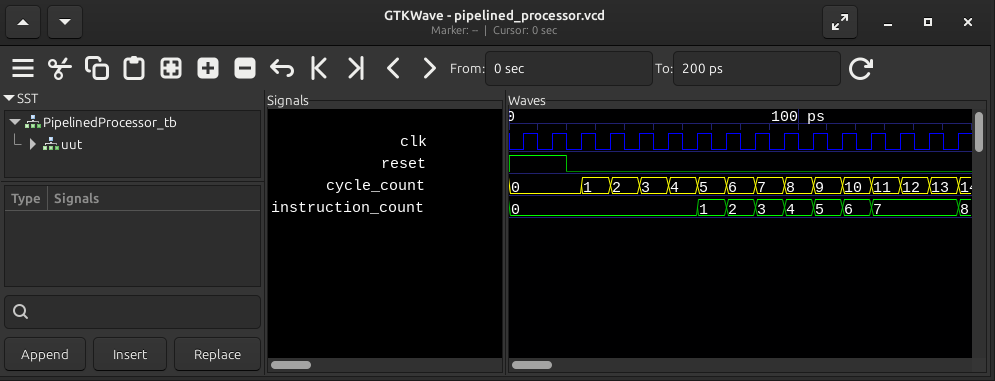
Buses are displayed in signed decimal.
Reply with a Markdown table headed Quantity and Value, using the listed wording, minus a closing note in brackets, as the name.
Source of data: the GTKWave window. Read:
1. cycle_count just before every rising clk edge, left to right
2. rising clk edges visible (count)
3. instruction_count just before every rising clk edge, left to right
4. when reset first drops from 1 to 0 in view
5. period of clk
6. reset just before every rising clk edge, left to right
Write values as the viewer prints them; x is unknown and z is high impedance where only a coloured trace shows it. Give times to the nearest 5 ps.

| Quantity | Value |
|---|---|
| cycle_count just before every rising clk edge, left to right | 0, 0, 0, 1, 2, 3, 4, 5, 6, 7, 8, 9, 10, 11, 12, 13 |
| rising clk edges visible | 16 |
| instruction_count just before every rising clk edge, left to right | 0, 0, 0, 0, 0, 0, 0, 1, 2, 3, 4, 5, 6, 7, 7, 7 |
| when reset first drops from 1 to 0 in view | 20 ps |
| period of clk | 10 ps |
| reset just before every rising clk edge, left to right | 1 1 0 0 0 0 0 0 0 0 0 0 0 0 0 0 |
